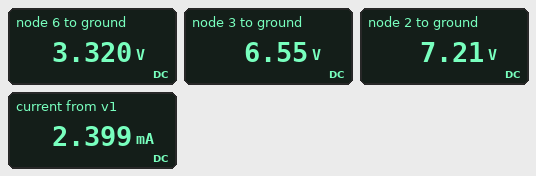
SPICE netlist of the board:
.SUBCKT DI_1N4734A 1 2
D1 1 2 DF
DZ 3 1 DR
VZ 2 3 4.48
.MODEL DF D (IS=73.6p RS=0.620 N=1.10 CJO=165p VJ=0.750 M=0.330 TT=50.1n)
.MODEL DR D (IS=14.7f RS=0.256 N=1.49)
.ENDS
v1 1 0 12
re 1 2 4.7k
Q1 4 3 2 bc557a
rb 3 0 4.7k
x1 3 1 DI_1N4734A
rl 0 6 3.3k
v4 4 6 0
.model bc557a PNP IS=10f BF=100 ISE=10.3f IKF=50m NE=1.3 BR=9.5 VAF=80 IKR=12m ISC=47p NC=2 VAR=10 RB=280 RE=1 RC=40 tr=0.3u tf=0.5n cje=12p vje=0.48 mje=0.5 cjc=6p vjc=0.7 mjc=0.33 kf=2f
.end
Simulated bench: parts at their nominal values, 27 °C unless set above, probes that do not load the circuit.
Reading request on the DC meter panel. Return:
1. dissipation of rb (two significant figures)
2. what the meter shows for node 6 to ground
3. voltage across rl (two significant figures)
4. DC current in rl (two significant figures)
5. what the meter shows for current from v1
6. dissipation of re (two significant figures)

9.1 mW
3.320 V
3.3 V
1.0 mA
2.399 mA
4.9 mW
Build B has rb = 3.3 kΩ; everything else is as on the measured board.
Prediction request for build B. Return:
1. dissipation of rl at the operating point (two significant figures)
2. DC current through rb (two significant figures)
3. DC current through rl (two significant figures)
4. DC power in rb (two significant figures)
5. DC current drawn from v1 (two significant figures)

3.4 mW
2.0 mA
1.0 mA
13 mW
3.0 mA
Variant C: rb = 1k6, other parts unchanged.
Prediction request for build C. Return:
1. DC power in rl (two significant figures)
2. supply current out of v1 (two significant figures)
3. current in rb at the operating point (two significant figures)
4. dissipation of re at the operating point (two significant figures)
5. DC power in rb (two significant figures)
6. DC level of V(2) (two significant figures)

3.4 mW
5.1 mA
4.1 mA
5.0 mW
26 mW
7.2 V
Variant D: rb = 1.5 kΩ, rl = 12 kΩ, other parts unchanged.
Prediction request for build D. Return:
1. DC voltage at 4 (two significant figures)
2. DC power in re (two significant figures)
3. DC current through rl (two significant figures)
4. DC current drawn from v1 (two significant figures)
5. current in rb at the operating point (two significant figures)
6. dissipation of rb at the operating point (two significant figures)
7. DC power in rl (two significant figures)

7.3 V
4.7 mW
610 µA
4.9 mA
4.3 mA
28 mW
4.4 mW
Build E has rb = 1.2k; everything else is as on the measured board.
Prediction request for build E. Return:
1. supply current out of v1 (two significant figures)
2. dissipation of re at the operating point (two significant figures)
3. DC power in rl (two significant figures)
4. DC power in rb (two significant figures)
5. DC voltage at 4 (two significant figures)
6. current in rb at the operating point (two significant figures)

6.4 mA
5.0 mW
3.4 mW
35 mW
3.4 V
5.4 mA
